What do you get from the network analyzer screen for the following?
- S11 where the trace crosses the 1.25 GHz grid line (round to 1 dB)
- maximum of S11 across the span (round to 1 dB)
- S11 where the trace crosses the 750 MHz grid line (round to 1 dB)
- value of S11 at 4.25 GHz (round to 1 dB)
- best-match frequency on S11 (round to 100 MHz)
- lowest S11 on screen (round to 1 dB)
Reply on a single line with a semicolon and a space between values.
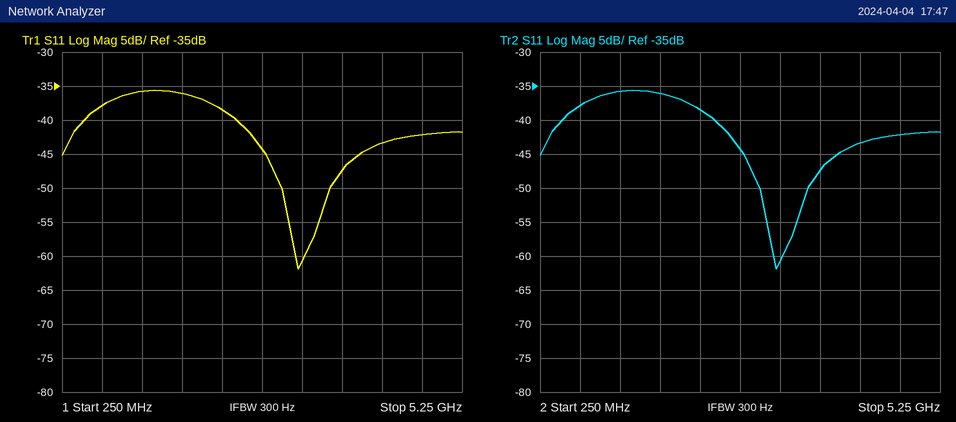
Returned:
-36 dB; -36 dB; -38 dB; -43 dB; 3.2 GHz; -62 dB
